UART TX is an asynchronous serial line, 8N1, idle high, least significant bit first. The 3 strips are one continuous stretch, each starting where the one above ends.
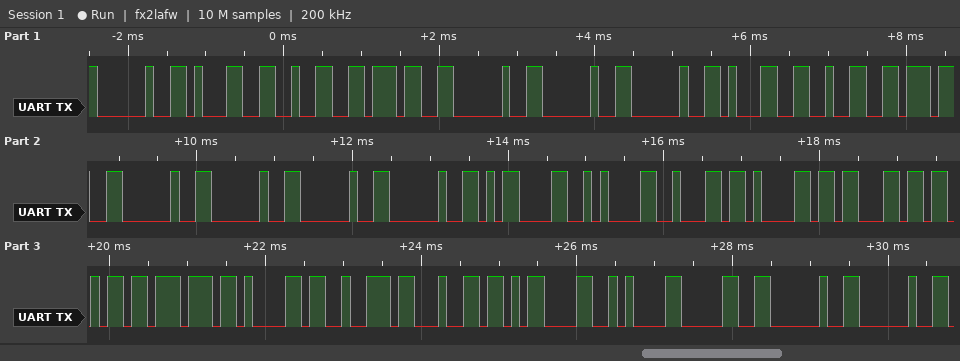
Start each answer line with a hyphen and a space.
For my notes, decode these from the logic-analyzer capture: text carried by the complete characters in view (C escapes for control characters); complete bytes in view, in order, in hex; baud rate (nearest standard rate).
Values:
- " 127   127    \r\nbackward\r\n0  "
- 20 31 32 37 20 20 20 31 32 37 20 20 20 20 0D 0A 62 61 63 6B 77 61 72 64 0D 0A 30 20 20
- 9600 baud
